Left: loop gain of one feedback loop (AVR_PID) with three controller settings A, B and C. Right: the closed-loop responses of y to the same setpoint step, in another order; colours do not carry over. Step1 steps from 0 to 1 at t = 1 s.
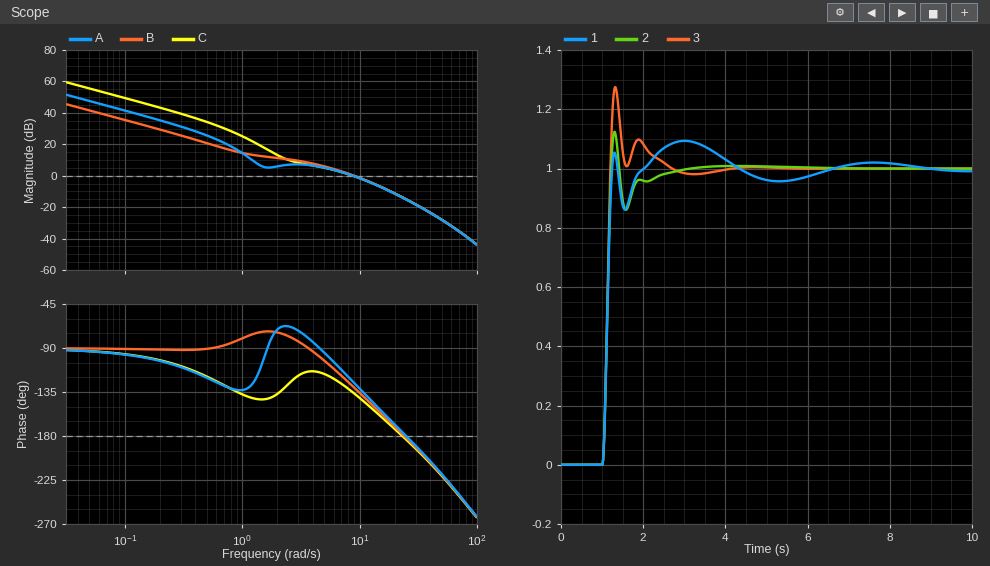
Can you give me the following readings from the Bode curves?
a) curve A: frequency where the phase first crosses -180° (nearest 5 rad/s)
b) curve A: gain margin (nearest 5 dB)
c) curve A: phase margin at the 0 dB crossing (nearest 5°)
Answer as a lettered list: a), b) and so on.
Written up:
a) 25 rad/s
b) 15 dB
c) 55°
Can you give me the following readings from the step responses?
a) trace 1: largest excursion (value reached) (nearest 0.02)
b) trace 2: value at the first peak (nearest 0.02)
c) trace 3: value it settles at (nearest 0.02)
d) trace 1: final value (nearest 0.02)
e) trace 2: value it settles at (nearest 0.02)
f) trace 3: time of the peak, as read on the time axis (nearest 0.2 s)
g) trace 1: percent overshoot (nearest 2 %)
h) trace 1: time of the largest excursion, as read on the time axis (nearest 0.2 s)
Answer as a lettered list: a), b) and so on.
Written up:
a) 1.10
b) 1.12
c) 1.00
d) 1.00
e) 1.00
f) 1.4 s
g) 10 %
h) 3.0 s
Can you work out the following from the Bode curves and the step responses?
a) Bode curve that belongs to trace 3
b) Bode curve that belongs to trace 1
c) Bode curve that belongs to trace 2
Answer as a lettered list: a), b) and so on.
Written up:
a) C
b) A
c) B
